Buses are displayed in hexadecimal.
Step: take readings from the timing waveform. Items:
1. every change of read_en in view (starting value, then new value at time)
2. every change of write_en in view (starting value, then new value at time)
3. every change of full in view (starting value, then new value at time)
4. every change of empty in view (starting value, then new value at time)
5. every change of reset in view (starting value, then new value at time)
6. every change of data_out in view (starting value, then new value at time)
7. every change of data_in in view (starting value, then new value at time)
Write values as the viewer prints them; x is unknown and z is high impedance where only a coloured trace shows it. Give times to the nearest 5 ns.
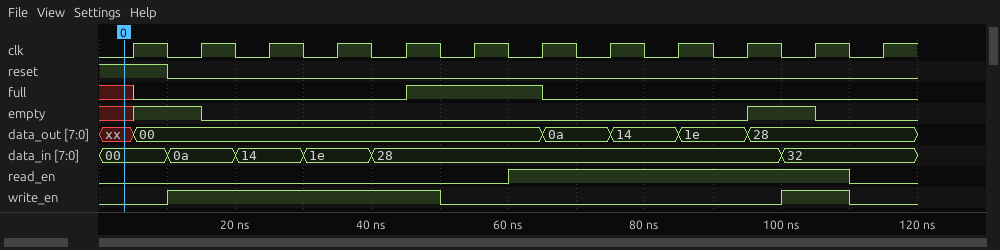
0, 1 at 60 ns, 0 at 110 ns
0, 1 at 10 ns, 0 at 50 ns, 1 at 100 ns, 0 at 110 ns
x, 0 at 5 ns, 1 at 45 ns, 0 at 65 ns
x, 1 at 5 ns, 0 at 15 ns, 1 at 95 ns, 0 at 105 ns
1, 0 at 10 ns
xx, 00 at 5 ns, 0a at 65 ns, 14 at 75 ns, 1e at 85 ns, 28 at 95 ns
00, 0a at 10 ns, 14 at 20 ns, 1e at 30 ns, 28 at 40 ns, 32 at 100 ns
